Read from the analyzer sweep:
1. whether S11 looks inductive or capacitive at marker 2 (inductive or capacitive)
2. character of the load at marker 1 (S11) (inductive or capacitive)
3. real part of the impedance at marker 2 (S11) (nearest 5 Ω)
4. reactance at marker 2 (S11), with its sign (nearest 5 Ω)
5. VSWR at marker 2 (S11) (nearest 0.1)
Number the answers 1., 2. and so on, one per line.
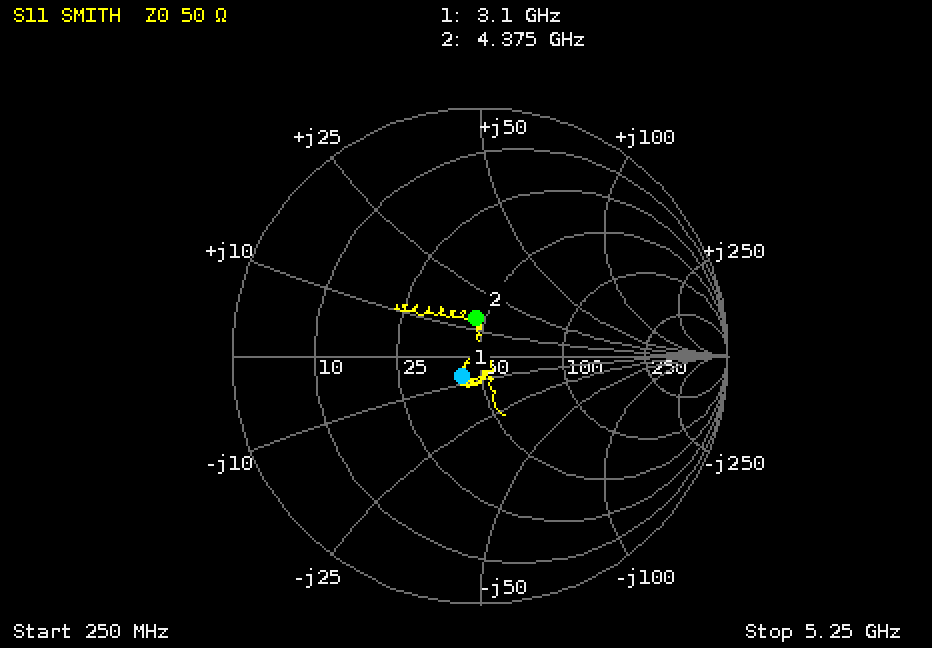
1. inductive
2. capacitive
3. 45 Ω
4. +15 Ω
5. 1.4
